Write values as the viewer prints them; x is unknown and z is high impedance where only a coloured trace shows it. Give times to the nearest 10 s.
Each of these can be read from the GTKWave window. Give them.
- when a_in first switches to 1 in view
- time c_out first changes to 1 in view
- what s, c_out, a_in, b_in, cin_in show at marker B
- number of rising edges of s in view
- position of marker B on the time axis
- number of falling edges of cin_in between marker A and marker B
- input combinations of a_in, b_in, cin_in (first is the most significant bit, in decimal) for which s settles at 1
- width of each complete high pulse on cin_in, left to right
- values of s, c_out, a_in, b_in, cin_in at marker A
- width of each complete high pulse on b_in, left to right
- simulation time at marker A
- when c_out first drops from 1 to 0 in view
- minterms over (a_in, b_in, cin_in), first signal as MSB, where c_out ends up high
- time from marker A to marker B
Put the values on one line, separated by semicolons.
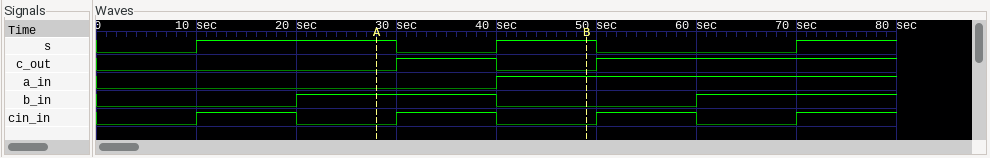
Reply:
40 s; 30 s; s=1, c_out=0, a_in=1, b_in=0, cin_in=0; 3; 50 s; 1; 1, 2, 4, 7; 10 s, 10 s, 10 s; s=1, c_out=0, a_in=0, b_in=1, cin_in=0; 20 s; 30 s; 40 s; 3, 5, 6, 7; 20 s
